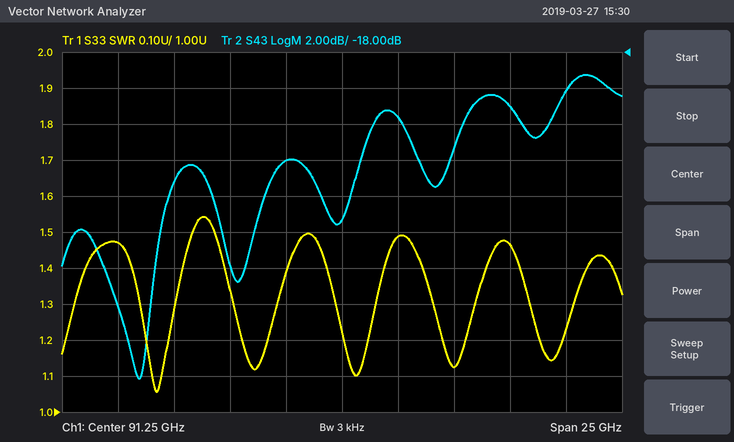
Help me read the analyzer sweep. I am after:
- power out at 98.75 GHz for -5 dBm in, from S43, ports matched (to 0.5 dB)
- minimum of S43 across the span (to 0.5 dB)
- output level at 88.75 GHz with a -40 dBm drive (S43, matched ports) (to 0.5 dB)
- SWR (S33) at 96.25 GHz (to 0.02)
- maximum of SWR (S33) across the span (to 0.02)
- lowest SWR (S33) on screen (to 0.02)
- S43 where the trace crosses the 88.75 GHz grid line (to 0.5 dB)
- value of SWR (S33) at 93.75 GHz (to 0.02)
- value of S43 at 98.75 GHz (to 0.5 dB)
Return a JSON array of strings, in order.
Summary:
["-26.0 dBm", "-36.0 dB", "-64.0 dBm", "1.12", "1.54", "1.06", "-24.0 dB", "1.48", "-21.0 dB"]
